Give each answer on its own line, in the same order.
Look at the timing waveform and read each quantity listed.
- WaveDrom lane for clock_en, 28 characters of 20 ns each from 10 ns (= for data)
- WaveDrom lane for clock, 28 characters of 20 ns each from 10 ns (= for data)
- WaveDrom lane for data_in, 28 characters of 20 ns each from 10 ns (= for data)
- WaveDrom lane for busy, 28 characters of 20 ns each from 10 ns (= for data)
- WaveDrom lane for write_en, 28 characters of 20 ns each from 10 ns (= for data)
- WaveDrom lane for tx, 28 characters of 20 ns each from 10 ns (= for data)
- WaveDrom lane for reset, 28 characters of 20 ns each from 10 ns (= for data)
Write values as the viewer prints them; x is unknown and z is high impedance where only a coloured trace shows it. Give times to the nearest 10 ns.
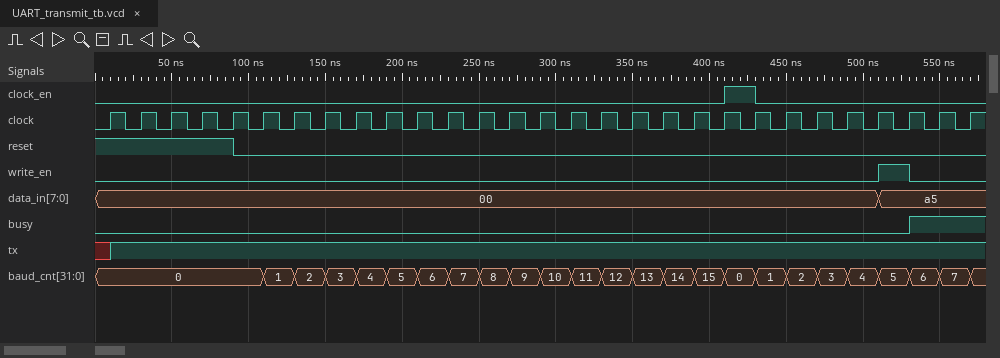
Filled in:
{name: 'clock_en', wave: '0...................10......'}
{name: 'clock', wave: 'p...........................'}
{name: 'data_in', wave: '=........................=..', data: '00 a5'}
{name: 'busy', wave: '0.........................1.'}
{name: 'write_en', wave: '0........................10.'}
{name: 'tx', wave: '1...........................'}
{name: 'reset', wave: '1...0.......................'}
